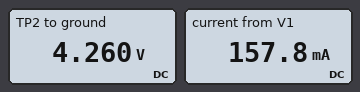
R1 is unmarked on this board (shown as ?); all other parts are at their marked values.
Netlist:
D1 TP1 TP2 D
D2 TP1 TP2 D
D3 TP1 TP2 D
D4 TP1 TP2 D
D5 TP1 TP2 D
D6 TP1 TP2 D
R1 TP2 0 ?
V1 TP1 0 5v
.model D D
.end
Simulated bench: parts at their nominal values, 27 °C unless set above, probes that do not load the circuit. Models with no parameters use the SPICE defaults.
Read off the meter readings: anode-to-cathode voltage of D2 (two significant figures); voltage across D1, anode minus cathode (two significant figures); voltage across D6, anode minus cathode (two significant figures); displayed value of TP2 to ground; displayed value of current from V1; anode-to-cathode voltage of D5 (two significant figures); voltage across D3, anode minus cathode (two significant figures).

740 mV
740 mV
740 mV
4.260 V
157.8 mA
740 mV
740 mV
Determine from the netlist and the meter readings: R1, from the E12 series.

27 Ω
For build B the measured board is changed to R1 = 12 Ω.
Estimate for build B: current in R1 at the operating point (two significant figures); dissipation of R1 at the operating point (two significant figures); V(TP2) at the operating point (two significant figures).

350 mA
1.5 W
4.2 V
